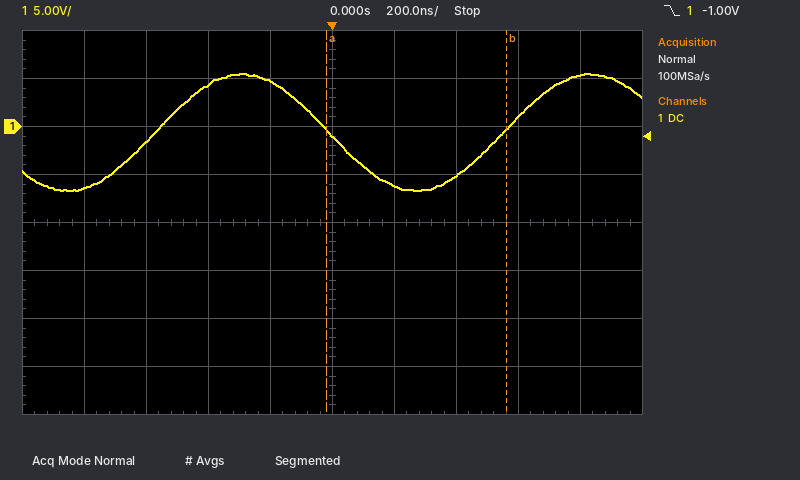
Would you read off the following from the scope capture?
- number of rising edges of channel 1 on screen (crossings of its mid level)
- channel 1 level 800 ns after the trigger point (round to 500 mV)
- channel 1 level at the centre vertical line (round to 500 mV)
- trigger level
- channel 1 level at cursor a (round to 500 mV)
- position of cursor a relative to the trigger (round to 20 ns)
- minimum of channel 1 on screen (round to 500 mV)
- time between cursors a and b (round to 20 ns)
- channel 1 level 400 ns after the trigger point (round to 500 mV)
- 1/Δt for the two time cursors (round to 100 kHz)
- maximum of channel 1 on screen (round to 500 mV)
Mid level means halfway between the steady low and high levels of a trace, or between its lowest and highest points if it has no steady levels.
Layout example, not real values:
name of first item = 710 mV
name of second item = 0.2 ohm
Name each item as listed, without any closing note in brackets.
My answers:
number of rising edges of channel 1 on screen = 2
channel 1 level 800 ns after the trigger point = 5.5 V
channel 1 level at the centre vertical line = -1.0 V
trigger level = -1.00 V
channel 1 level at cursor a = -500 mV
position of cursor a relative to the trigger = -20 ns
minimum of channel 1 on screen = -6.5 V
time between cursors a and b = 580 ns
channel 1 level 400 ns after the trigger point = -5.0 V
1/Δt for the two time cursors = 1.7 MHz
maximum of channel 1 on screen = 5.5 V
